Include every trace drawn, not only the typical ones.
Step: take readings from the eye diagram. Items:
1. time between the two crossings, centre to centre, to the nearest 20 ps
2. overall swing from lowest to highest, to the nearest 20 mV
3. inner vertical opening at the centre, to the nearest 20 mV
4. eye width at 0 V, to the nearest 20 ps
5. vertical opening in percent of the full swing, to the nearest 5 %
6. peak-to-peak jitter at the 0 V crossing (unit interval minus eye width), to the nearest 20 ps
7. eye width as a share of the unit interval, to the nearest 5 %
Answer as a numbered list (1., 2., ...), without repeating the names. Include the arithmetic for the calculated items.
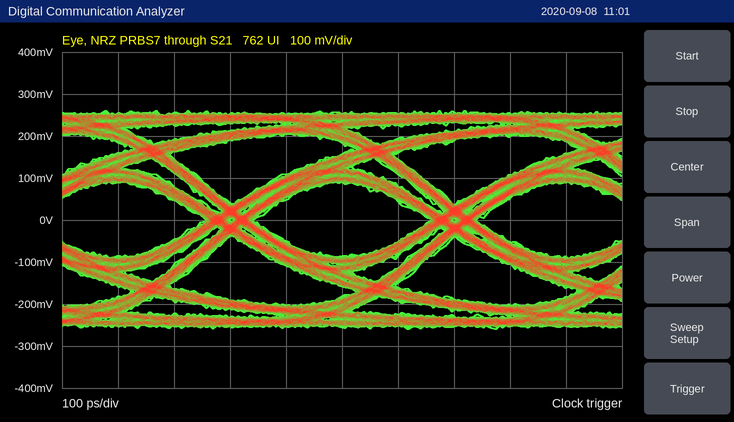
1. 400 ps
2. 520 mV
3. 180 mV
4. 320 ps
5. 180 mV / 520 mV ≈ 35 %
6. 80 ps
7. 320 ps / 400 ps ≈ 80 %
